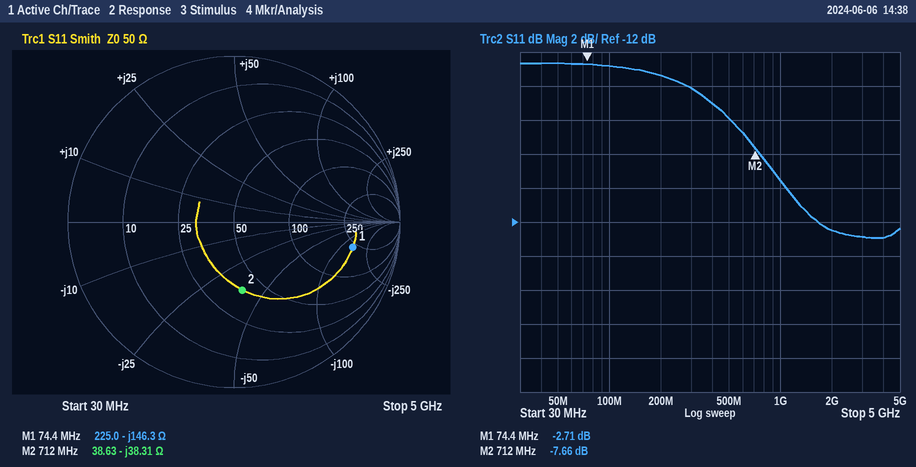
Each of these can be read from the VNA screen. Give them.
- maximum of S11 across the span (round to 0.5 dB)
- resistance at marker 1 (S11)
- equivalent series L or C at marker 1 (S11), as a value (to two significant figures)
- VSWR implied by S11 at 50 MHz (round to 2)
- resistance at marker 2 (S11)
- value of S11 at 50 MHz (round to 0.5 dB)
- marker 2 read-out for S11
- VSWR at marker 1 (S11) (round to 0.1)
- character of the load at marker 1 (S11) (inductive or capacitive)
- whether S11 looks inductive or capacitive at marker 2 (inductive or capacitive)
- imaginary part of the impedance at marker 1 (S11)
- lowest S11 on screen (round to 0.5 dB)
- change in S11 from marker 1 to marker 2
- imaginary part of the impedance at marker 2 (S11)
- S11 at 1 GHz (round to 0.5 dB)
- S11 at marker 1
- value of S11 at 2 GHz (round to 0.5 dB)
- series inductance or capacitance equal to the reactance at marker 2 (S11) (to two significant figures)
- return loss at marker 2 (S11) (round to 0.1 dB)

-2.5 dB
225.0 Ω
15 pF
6
38.63 Ω
-2.5 dB
-7.66 dB
6.5
capacitive
capacitive
-146.3 Ω
-13.0 dB
-4.95 dB
-38.31 Ω
-9.5 dB
-2.71 dB
-12.5 dB
5.8 pF
7.7 dB
